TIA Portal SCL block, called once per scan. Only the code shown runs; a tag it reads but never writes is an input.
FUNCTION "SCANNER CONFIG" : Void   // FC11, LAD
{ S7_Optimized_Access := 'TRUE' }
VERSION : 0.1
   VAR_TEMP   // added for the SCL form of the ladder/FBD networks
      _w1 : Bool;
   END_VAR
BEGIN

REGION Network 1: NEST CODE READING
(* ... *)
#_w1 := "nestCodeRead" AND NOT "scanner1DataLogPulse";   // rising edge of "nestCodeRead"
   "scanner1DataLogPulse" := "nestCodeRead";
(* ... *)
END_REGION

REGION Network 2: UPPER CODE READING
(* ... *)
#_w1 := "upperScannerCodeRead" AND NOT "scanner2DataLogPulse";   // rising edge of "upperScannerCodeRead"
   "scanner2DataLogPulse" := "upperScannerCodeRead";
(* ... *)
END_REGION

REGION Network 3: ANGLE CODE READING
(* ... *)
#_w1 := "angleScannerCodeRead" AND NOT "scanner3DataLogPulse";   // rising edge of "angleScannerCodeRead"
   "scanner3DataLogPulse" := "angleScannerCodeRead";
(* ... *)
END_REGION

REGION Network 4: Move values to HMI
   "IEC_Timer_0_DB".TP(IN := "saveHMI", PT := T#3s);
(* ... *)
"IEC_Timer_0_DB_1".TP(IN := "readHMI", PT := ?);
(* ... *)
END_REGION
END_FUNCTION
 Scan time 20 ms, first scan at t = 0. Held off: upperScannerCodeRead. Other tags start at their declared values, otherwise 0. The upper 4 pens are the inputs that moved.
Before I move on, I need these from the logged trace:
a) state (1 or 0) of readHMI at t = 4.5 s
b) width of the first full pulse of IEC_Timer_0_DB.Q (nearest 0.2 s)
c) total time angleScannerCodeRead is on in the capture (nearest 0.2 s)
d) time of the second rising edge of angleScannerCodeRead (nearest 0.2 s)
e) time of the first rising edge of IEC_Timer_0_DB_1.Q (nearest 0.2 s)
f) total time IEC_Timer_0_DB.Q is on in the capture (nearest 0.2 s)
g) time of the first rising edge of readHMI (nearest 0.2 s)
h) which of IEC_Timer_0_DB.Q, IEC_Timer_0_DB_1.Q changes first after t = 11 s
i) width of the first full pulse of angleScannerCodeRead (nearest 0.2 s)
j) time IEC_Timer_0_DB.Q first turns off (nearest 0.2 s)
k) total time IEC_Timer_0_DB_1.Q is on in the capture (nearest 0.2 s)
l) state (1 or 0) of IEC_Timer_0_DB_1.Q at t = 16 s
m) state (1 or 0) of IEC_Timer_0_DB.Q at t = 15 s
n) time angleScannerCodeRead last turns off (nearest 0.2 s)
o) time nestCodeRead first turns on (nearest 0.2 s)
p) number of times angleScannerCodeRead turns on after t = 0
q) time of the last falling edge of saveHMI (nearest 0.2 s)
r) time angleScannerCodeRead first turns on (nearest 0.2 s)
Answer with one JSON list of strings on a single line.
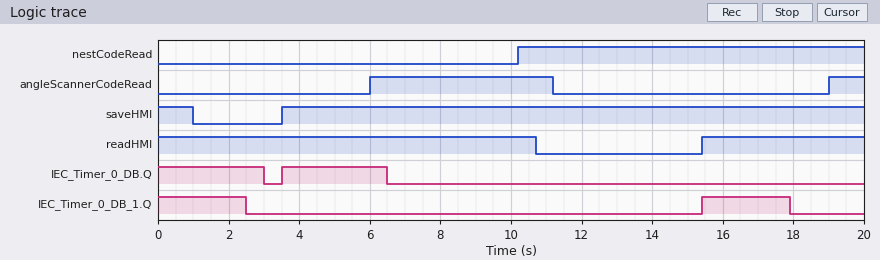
["1", "3.0 s", "6.2 s", "19.0 s", "15.4 s", "6.0 s", "15.4 s", "IEC_Timer_0_DB_1.Q", "5.2 s", "3.0 s", "5.0 s", "1", "0", "11.2 s", "10.2 s", "2", "1.0 s", "6.0 s"]
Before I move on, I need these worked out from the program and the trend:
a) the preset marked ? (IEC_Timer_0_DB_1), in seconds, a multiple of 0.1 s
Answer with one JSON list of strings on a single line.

["2.5 s"]
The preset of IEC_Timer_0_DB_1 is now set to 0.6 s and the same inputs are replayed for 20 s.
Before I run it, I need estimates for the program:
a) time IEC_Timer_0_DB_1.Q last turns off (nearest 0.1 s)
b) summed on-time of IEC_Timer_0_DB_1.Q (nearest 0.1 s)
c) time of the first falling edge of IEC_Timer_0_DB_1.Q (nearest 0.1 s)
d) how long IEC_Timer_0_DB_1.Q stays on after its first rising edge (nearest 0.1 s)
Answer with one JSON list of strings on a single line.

["16.0 s", "1.2 s", "0.6 s", "0.6 s"]
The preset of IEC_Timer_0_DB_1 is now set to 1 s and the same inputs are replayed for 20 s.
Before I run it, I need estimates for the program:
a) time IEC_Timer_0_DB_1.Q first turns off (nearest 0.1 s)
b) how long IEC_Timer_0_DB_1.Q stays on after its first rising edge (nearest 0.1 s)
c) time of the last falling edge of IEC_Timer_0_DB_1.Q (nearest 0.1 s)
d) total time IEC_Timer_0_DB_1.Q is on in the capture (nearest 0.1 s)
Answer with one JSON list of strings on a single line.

["1.0 s", "1.0 s", "16.4 s", "2.0 s"]
